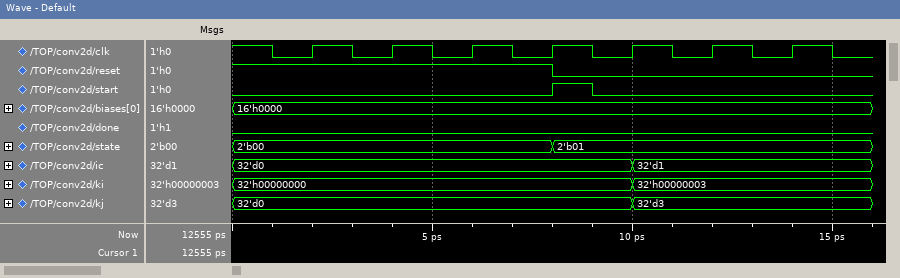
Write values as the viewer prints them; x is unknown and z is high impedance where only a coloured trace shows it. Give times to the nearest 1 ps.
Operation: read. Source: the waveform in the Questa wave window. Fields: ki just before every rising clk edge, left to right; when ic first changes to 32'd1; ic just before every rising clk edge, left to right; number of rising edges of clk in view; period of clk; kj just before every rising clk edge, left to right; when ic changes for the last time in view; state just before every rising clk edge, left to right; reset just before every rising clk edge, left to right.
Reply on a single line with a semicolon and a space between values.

32'h00000000, 32'h00000000, 32'h00000000, 32'h00000000, 32'h00000000, 32'h00000003, 32'h00000003; 10 ps; 32'd0, 32'd0, 32'd0, 32'd0, 32'd0, 32'd1, 32'd1; 7; 2 ps; 32'd0, 32'd0, 32'd0, 32'd0, 32'd0, 32'd3, 32'd3; 10 ps; 2'b00, 2'b00, 2'b00, 2'b00, 2'b01, 2'b01, 2'b01; 1 1 1 1 0 0 0
